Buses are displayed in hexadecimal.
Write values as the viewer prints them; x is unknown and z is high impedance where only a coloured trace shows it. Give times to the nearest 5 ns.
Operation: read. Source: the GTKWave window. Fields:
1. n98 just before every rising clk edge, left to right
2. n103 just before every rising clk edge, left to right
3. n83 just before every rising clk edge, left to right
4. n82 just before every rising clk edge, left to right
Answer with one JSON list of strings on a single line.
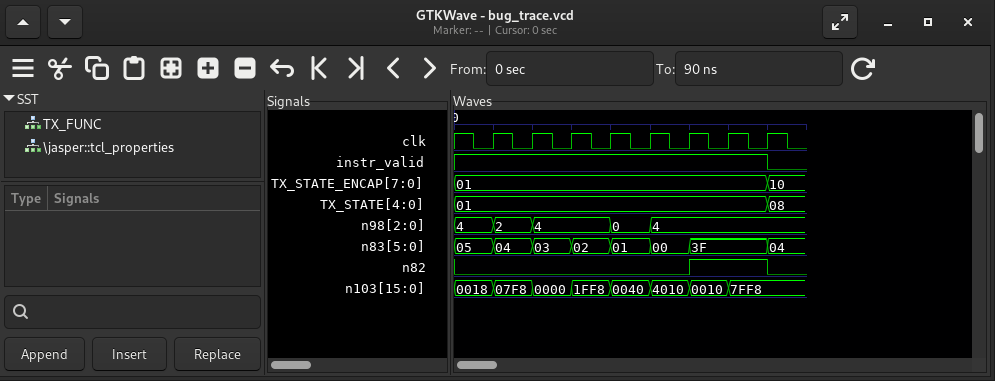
["4, 2, 4, 4, 0, 4, 4, 4", "0018, 07F8, 0000, 1FF8, 0040, 4010, 0010, 7FF8", "05, 04, 03, 02, 01, 00, 3F, 3F", "0 0 0 0 0 0 1 1"]
